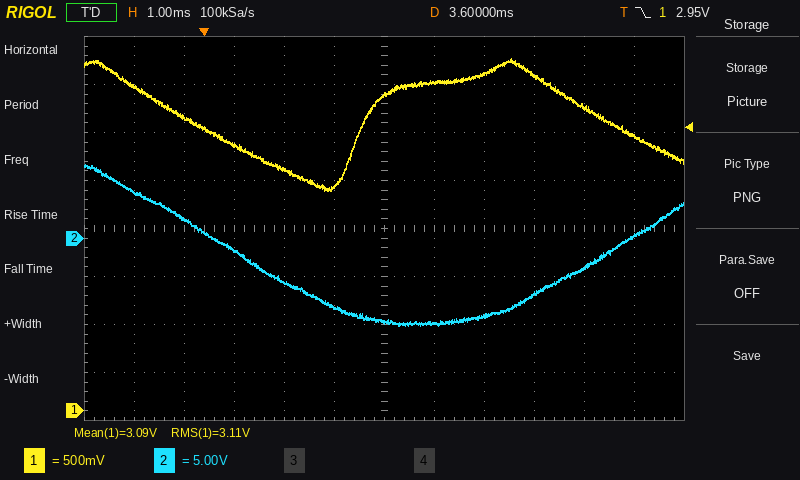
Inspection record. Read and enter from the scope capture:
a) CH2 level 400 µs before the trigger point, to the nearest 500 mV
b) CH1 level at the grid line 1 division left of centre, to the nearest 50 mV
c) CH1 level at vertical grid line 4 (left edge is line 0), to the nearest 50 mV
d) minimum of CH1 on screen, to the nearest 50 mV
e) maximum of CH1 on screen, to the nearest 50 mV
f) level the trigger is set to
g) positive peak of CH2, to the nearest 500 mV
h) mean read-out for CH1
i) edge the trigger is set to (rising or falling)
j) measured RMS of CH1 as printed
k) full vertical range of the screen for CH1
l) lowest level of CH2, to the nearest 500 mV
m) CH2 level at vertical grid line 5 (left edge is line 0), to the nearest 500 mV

2.0 V
2.35 V
2.50 V
2.30 V
3.65 V
2.95 V
7.5 V
3.09 V
falling
3.11 V
4 V
-9.0 V
-7.0 V
